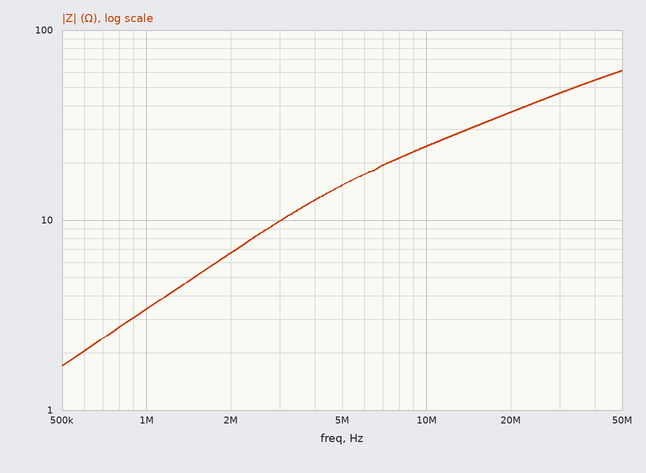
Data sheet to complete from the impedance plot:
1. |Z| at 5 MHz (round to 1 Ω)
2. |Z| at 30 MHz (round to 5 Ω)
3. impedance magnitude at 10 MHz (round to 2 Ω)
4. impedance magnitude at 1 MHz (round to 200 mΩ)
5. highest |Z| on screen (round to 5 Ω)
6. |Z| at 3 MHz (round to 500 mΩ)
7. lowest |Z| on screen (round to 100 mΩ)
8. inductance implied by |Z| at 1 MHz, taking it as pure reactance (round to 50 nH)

15 Ω
45 Ω
24 Ω
3.4 Ω
60 Ω
10.0 Ω
1.7 Ω
550 nH
